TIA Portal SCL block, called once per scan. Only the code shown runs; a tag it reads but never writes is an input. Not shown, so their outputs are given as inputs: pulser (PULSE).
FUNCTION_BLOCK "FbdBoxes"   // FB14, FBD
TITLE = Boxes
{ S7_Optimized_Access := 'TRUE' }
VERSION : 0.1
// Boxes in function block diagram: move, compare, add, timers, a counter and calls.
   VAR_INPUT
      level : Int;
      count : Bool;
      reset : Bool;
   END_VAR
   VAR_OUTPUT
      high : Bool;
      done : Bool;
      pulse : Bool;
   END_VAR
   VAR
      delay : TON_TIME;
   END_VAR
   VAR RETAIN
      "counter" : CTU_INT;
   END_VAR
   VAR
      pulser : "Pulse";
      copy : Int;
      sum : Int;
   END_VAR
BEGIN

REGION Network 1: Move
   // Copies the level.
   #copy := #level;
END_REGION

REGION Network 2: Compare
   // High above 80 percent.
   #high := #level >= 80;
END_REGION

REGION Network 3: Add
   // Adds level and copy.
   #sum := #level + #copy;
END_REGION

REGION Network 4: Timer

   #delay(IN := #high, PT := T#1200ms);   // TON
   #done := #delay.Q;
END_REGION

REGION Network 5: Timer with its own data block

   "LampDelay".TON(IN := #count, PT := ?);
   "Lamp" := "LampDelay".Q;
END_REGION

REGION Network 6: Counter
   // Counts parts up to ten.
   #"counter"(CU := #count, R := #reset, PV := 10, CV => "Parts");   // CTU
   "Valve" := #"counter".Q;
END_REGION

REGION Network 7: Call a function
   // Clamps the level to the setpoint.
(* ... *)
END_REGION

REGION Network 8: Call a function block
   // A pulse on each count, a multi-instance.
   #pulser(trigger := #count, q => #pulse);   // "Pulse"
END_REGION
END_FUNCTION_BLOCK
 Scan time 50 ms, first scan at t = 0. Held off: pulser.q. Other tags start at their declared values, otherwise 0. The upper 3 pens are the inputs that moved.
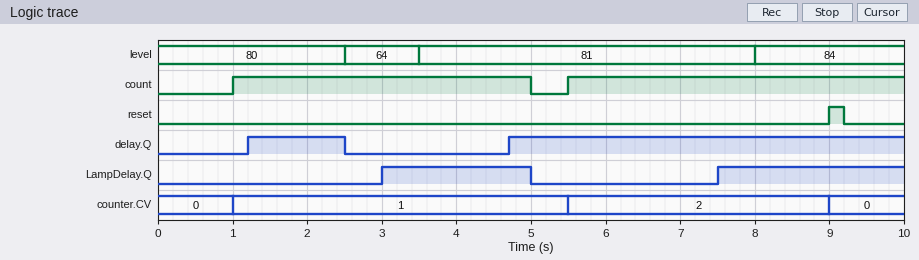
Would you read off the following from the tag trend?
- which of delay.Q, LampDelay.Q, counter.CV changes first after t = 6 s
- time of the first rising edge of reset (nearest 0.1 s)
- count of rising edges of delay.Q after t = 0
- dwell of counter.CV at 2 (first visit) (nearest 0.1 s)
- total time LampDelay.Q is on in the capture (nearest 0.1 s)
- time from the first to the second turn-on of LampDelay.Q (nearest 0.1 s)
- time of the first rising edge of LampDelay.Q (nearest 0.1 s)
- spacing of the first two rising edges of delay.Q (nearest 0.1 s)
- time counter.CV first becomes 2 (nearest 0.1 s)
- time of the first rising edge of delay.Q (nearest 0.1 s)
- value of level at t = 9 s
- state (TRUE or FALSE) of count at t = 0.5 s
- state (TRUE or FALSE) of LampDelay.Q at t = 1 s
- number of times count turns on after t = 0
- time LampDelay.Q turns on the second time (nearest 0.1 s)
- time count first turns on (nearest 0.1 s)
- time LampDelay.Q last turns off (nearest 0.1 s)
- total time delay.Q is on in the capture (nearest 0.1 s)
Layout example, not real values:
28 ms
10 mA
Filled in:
LampDelay.Q
9.0 s
2
3.5 s
4.5 s
4.5 s
3.0 s
3.5 s
5.5 s
1.2 s
84
FALSE
FALSE
2
7.5 s
1.0 s
5.0 s
6.6 s
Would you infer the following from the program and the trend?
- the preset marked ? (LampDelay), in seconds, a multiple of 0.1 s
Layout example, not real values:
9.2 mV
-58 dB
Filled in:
2.0 s
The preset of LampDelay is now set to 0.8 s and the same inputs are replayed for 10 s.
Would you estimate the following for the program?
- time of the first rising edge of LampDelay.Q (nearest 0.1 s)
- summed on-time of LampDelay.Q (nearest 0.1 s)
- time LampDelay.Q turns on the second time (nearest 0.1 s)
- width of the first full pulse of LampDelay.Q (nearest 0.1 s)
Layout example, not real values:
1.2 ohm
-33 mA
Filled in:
1.8 s
6.9 s
6.3 s
3.2 s
